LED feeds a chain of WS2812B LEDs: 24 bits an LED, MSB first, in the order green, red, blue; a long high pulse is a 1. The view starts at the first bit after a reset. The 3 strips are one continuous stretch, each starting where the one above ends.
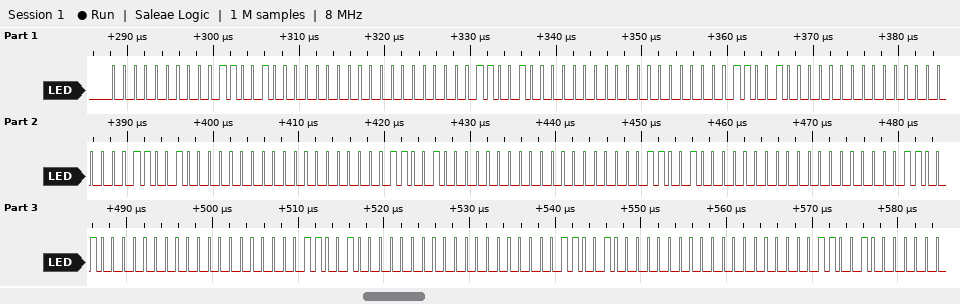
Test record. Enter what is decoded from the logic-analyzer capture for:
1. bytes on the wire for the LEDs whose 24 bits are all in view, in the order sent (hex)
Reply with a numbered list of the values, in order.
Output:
1. 00 32 00 00 32 00 00 32 00 00 32 00 00 32 00 00 32 00 00 32 00 00 32 00 00 32 00
